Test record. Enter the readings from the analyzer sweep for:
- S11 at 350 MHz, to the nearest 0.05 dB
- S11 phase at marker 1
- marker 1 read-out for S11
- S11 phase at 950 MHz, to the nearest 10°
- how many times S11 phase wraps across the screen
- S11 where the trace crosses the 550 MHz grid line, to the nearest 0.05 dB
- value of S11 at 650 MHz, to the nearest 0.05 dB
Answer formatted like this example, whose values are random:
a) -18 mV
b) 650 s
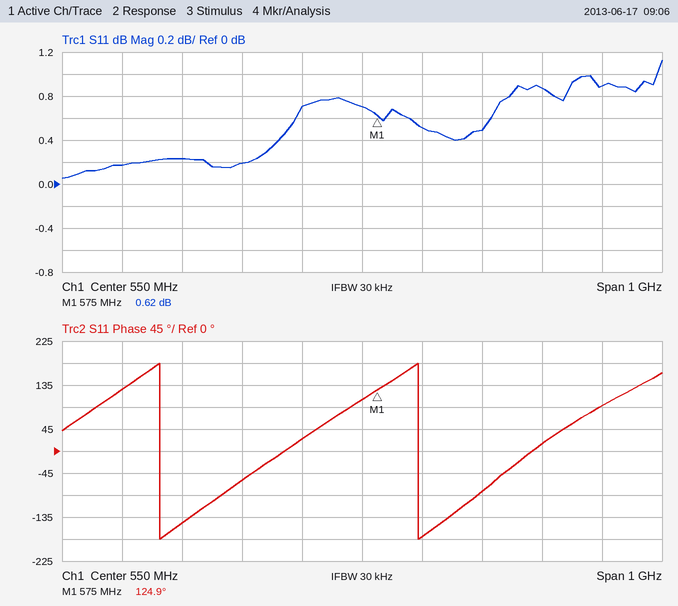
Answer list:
a) 0.20 dB
b) 124.9°
c) 0.62 dB
d) 90°
e) 2
f) 0.70 dB
g) 0.50 dB
